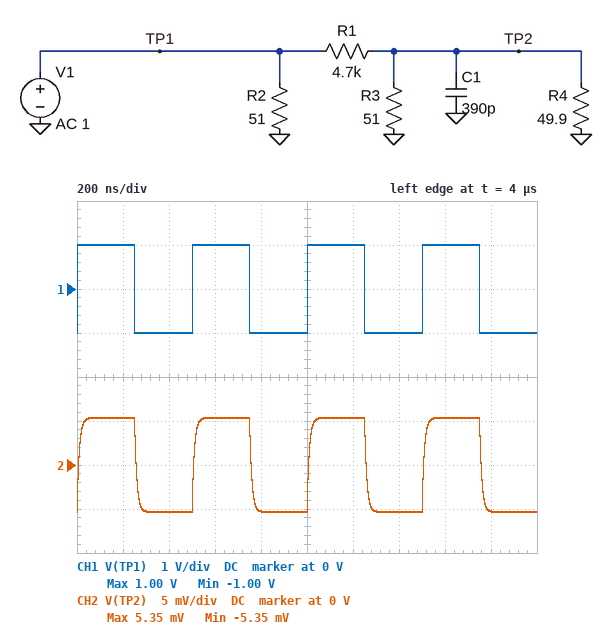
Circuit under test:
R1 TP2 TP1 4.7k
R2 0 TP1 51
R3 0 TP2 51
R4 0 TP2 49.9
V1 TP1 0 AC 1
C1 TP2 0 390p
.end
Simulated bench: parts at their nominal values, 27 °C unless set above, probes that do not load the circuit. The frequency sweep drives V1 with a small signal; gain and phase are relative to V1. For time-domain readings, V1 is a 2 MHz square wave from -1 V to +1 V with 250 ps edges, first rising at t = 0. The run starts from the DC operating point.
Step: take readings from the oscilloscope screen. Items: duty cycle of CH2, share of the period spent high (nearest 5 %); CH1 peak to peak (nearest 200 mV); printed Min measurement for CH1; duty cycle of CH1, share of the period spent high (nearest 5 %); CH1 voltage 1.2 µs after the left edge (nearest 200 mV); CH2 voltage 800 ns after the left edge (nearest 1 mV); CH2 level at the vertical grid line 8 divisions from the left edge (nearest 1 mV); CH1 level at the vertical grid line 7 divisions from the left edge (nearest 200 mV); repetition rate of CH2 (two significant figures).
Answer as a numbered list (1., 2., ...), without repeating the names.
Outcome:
1. 50 %
2. 2.0 V
3. -1.00 V
4. 50 %
5. 1.0 V
6. -5 mV
7. 5 mV
8. -1.0 V
9. 2.0 MHz
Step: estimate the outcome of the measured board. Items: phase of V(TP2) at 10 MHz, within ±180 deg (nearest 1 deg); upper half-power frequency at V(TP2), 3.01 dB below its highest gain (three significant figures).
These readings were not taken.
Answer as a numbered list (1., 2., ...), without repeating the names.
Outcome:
1. -32 deg
2. 16.3 MHz
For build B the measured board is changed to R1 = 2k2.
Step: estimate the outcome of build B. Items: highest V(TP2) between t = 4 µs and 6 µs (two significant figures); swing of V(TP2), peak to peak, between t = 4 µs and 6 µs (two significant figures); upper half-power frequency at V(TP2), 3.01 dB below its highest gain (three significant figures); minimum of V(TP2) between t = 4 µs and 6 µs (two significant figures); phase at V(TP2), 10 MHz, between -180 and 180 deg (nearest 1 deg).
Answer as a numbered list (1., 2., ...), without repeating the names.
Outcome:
1. 11 mV
2. 23 mV
3. 16.4 MHz
4. -11 mV
5. -31 deg
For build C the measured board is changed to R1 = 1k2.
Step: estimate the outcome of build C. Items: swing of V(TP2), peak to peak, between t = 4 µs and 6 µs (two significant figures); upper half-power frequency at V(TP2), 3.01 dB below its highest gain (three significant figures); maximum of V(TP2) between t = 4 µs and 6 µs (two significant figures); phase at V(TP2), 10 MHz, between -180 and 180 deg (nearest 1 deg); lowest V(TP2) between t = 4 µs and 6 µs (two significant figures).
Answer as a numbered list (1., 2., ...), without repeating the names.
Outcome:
1. 41 mV
2. 16.5 MHz
3. 21 mV
4. -31 deg
5. -21 mV
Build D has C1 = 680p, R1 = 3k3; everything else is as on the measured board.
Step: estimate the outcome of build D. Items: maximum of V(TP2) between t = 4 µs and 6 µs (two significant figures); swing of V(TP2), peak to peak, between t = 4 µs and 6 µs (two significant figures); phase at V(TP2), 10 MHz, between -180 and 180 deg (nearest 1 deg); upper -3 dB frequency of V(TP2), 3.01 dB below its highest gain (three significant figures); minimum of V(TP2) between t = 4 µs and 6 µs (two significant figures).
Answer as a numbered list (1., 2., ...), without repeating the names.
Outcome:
1. 7.6 mV
2. 15 mV
3. -47 deg
4. 9.35 MHz
5. -7.6 mV
